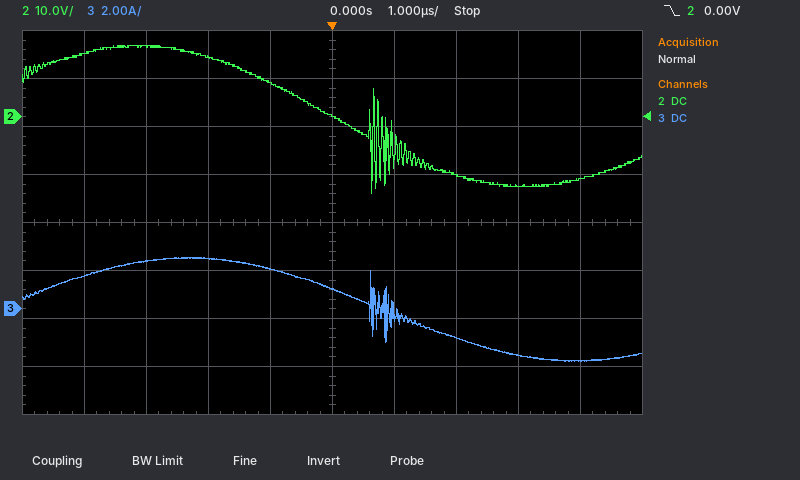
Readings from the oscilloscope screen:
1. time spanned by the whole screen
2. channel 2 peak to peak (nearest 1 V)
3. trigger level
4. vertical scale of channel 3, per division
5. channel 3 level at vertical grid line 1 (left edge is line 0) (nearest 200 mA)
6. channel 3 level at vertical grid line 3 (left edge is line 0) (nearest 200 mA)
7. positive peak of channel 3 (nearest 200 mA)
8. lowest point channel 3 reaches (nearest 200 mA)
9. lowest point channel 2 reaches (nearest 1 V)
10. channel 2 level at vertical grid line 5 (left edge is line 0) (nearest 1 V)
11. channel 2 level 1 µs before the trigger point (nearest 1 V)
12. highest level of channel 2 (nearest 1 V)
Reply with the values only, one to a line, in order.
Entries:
10 µs
31 V
0.00 V
2 A
1.4 A
2.0 A
2.2 A
-2.2 A
-16 V
0 V
7 V
15 V
